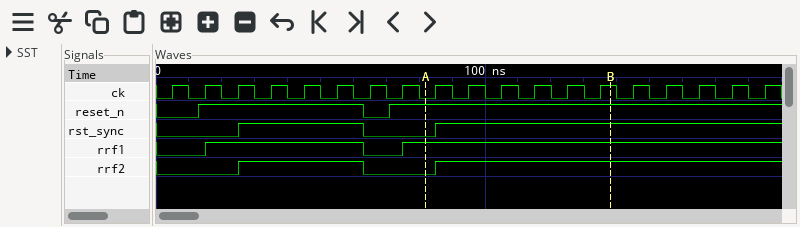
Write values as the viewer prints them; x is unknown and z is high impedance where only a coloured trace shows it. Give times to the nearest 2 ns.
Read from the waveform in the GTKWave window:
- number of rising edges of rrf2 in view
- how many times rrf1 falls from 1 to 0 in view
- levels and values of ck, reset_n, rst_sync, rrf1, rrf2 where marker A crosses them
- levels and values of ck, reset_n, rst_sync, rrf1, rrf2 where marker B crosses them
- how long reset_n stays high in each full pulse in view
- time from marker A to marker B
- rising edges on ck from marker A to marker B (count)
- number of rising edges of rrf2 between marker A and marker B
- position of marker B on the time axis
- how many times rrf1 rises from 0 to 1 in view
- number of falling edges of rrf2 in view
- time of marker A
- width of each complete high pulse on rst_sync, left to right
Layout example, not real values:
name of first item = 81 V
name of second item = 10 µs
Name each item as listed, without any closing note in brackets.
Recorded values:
number of rising edges of rrf2 in view = 2
how many times rrf1 falls from 1 to 0 in view = 1
levels and values of ck, reset_n, rst_sync, rrf1, rrf2 where marker A crosses them = ck=0, reset_n=1, rst_sync=0, rrf1=1, rrf2=0
levels and values of ck, reset_n, rst_sync, rrf1, rrf2 where marker B crosses them = ck=1, reset_n=1, rst_sync=1, rrf1=1, rrf2=1
how long reset_n stays high in each full pulse in view = 50 ns
time from marker A to marker B = 56 ns
rising edges on ck from marker A to marker B = 6
number of rising edges of rrf2 between marker A and marker B = 1
position of marker B on the time axis = 138 ns
how many times rrf1 rises from 0 to 1 in view = 2
number of falling edges of rrf2 in view = 1
time of marker A = 82 ns
width of each complete high pulse on rst_sync, left to right = 38 ns
